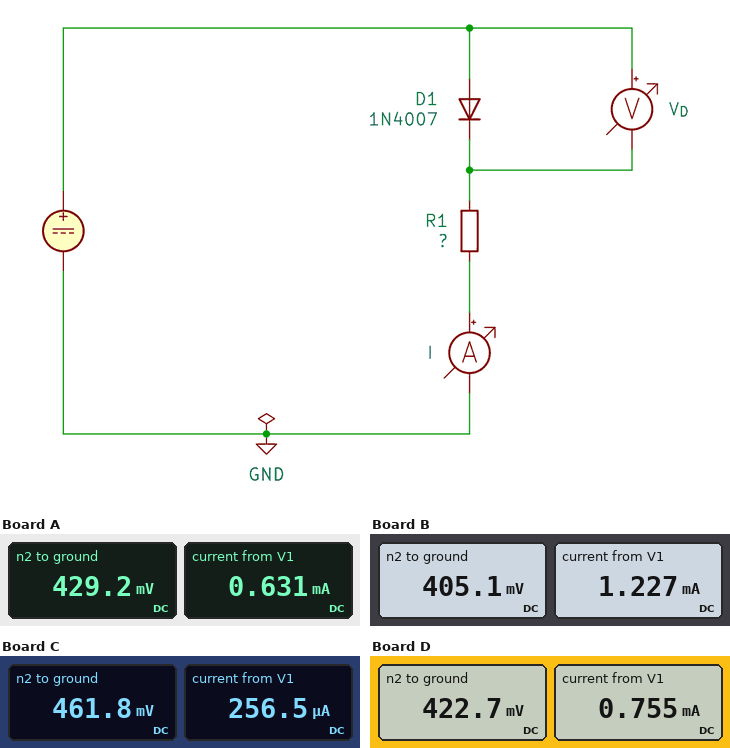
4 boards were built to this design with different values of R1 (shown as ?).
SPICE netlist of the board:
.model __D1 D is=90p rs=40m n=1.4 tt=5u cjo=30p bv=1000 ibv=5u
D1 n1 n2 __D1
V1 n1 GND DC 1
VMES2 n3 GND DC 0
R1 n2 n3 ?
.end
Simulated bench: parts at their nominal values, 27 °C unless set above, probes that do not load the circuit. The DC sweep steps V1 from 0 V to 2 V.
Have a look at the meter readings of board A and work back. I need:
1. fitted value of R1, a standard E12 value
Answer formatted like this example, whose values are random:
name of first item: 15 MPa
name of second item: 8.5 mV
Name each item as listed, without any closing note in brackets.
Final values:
fitted value of R1, a standard E12 value: 680 Ω
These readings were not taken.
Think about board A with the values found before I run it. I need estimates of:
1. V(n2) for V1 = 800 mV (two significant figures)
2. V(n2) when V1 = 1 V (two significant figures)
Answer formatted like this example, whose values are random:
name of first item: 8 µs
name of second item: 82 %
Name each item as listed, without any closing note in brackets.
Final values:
V(n2) for V1 = 800 mV: 250 mV
V(n2) when V1 = 1 V: 430 mV
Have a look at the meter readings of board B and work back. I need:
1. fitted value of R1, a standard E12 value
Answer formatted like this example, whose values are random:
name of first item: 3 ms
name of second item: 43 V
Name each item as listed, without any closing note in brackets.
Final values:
fitted value of R1, a standard E12 value: 330 Ω
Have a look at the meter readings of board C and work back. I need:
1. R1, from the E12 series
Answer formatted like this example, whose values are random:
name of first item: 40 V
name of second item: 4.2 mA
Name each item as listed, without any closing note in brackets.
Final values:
R1, from the E12 series: 1.8 kΩ
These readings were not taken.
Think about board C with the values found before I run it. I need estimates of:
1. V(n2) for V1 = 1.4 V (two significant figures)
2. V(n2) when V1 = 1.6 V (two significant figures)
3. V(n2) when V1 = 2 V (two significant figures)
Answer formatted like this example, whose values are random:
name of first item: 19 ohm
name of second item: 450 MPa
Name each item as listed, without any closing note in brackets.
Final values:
V(n2) for V1 = 1.4 V: 840 mV
V(n2) when V1 = 1.6 V: 1.0 V
V(n2) when V1 = 2 V: 1.4 V
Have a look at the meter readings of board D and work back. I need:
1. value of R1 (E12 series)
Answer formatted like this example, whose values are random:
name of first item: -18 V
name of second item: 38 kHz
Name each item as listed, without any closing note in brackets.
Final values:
value of R1: 560 Ω
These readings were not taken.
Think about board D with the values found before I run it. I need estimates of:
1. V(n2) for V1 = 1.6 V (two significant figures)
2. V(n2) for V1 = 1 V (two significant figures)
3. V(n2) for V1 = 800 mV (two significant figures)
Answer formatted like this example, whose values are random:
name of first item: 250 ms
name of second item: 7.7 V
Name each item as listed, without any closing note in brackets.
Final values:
V(n2) for V1 = 1.6 V: 990 mV
V(n2) for V1 = 1 V: 420 mV
V(n2) for V1 = 800 mV: 240 mV
